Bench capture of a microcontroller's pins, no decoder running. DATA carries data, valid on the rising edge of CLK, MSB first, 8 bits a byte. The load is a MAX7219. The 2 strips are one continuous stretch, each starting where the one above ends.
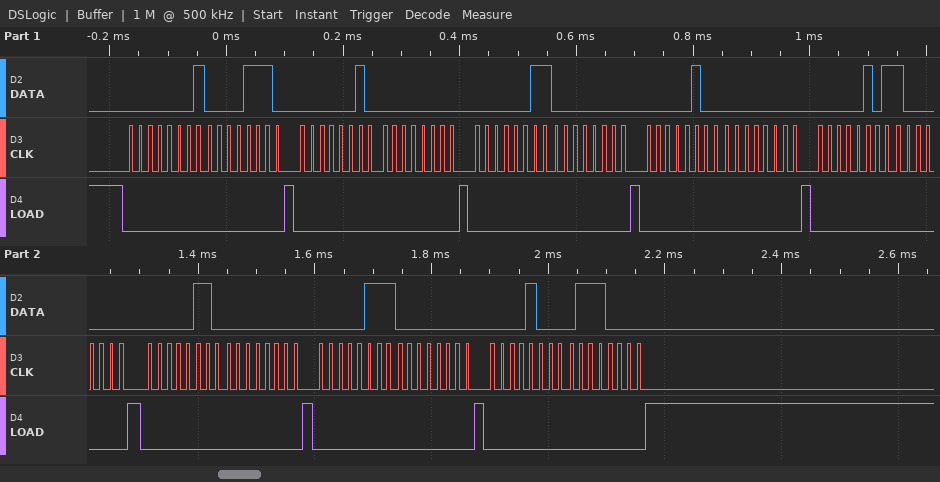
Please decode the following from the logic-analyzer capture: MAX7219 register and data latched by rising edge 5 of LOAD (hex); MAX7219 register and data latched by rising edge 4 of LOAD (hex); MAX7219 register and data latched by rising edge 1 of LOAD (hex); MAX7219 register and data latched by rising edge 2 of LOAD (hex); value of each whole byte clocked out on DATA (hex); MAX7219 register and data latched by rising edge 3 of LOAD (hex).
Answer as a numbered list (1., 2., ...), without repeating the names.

1. register 0x5, data 0x80
2. register 0x4, data 0x00
3. register 0x1, data 0x0E
4. register 0x2, data 0x00
5. 01 0E 02 00 03 00 04 00 05 80 06 00 07 00 08 70
6. register 0x3, data 0x00
